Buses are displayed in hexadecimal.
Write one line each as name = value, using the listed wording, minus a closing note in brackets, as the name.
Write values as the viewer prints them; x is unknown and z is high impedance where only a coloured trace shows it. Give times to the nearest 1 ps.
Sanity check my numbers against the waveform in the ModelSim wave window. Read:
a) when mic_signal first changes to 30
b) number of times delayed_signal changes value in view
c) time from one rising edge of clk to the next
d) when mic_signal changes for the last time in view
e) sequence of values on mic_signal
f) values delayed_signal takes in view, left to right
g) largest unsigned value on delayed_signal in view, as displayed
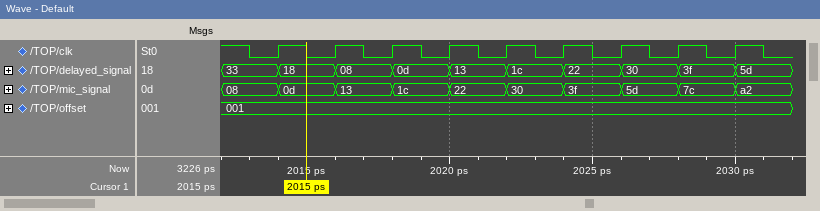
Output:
when mic_signal first changes to 30 = 2022 ps
number of times delayed_signal changes value in view = 9
time from one rising edge of clk to the next = 2 ps
when mic_signal changes for the last time in view = 2030 ps
sequence of values on mic_signal = 08, 0d, 13, 1c, 22, 30, 3f, 5d, 7c, a2
values delayed_signal takes in view, left to right = 33, 18, 08, 0d, 13, 1c, 22, 30, 3f, 5d
largest unsigned value on delayed_signal in view, as displayed = 5d
